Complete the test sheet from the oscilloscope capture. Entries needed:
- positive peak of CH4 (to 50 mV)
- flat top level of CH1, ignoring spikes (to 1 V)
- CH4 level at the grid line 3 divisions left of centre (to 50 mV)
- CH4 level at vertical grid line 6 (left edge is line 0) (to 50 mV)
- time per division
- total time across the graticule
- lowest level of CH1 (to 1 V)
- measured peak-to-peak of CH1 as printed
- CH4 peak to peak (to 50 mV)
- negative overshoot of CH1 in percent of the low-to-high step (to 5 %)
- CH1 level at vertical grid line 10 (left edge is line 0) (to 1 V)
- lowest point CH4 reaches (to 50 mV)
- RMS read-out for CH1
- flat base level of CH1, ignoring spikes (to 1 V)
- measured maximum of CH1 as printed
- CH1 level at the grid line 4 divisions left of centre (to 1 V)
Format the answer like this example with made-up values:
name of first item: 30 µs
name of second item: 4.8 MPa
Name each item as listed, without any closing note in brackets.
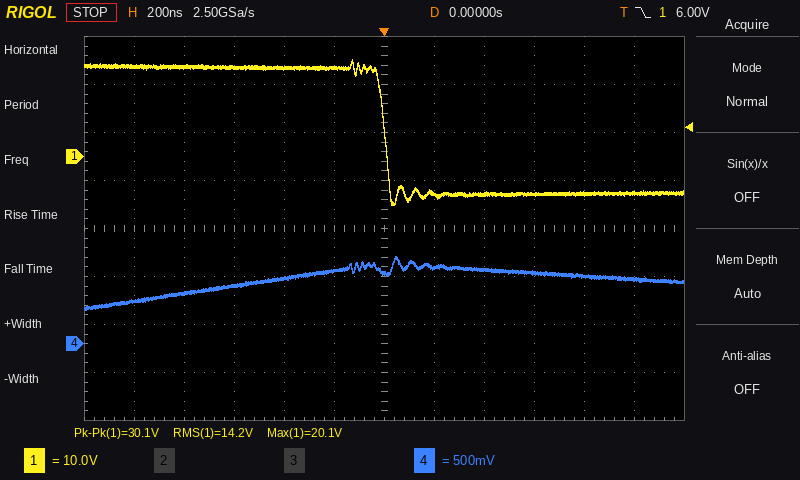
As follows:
positive peak of CH4: 900 mV
flat top level of CH1, ignoring spikes: 19 V
CH4 level at the grid line 3 divisions left of centre: 600 mV
CH4 level at vertical grid line 6 (left edge is line 0): 750 mV
time per division: 200 ns
total time across the graticule: 2.4 µs
lowest level of CH1: -10 V
measured peak-to-peak of CH1 as printed: 30.1 V
CH4 peak to peak: 550 mV
negative overshoot of CH1 in percent of the low-to-high step: 10 %
CH1 level at vertical grid line 10 (left edge is line 0): -8 V
lowest point CH4 reaches: 350 mV
RMS read-out for CH1: 14.2 V
flat base level of CH1, ignoring spikes: -8 V
measured maximum of CH1 as printed: 20.1 V
CH1 level at the grid line 4 divisions left of centre: 19 V
